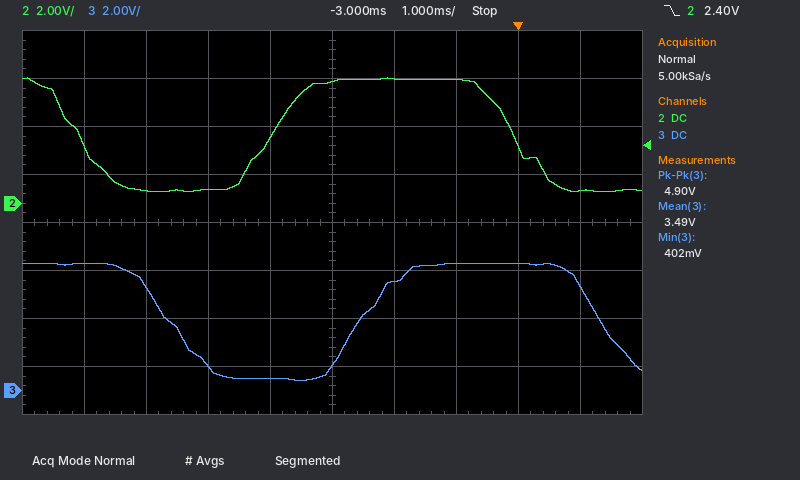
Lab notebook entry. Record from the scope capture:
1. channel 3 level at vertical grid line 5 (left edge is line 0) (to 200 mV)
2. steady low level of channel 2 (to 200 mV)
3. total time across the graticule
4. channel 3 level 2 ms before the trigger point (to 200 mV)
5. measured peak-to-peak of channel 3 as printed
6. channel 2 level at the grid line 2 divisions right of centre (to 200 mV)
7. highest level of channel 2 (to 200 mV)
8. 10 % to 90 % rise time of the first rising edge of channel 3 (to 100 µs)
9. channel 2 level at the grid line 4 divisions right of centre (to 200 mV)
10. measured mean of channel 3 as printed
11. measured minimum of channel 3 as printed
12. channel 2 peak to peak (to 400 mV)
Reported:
1.0 V
600 mV
10 ms
4.6 V
4.90 V
5.2 V
5.2 V
1.2 ms
600 mV
3.49 V
402 mV
4.8 V
